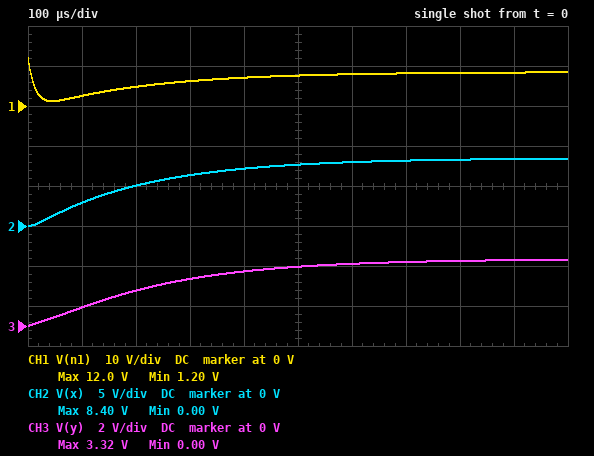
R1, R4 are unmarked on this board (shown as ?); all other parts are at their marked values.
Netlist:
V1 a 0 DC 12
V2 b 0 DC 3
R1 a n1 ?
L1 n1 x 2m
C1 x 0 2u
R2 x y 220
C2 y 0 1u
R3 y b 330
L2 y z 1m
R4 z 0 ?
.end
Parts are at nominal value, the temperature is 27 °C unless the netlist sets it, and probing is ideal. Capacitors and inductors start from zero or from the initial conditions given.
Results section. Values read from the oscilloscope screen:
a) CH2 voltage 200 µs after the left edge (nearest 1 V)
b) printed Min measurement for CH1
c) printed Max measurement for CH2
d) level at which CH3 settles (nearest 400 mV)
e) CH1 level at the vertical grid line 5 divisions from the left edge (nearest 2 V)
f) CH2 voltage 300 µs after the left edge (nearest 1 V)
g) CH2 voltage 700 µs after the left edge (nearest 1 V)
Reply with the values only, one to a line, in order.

5 V
1.20 V
8.40 V
3.2 V
8 V
6 V
8 V
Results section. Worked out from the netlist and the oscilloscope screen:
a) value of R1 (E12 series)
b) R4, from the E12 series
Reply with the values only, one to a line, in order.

150 Ω
150 Ω
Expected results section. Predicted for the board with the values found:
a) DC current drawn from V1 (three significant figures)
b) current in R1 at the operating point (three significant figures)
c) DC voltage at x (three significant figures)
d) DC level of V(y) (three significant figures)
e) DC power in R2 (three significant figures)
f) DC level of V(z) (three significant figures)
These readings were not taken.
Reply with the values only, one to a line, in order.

23.4 mA
23.4 mA
8.49 V
3.35 V
120 mW
3.35 V
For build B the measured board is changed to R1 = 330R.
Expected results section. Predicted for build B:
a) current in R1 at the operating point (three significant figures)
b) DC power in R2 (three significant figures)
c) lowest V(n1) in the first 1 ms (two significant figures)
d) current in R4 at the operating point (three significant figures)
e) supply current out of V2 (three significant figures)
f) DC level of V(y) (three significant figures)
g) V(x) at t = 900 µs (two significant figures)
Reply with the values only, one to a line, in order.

16.9 mA
63.1 mW
410 mV
17.9 mA
957 µA
2.68 V
5.9 V
